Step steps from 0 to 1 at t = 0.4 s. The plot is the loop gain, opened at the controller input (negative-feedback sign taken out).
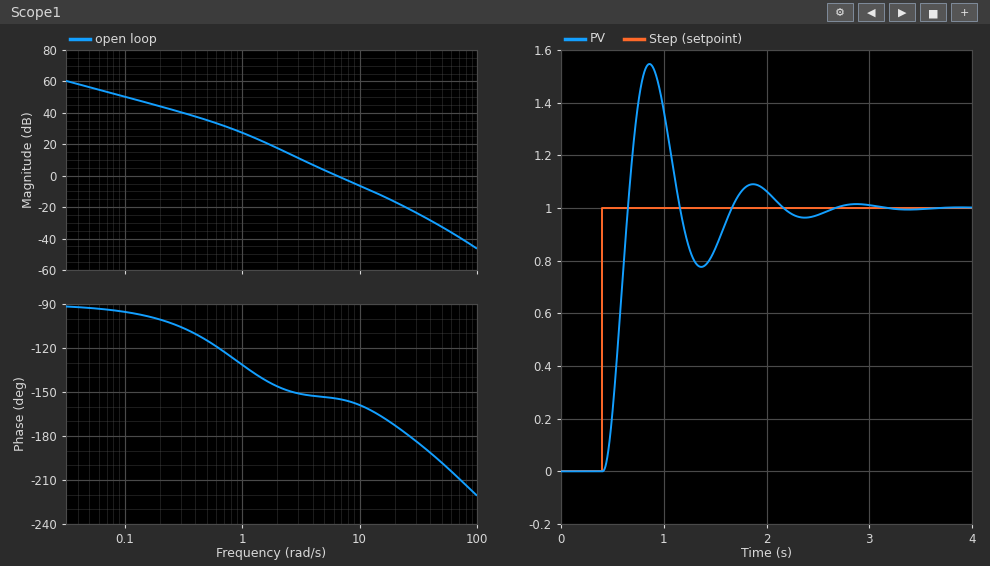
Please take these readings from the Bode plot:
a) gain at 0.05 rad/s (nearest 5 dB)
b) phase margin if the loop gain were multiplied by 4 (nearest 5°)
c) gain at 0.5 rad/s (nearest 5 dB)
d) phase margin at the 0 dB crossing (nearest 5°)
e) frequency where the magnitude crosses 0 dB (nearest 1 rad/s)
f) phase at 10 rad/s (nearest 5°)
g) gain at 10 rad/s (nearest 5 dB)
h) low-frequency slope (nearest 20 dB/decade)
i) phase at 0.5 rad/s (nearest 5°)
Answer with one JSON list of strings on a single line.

["55 dB", "15°", "35 dB", "25°", "6 rad/s", "-160°", "-5 dB", "-20 dB/decade", "-115°"]
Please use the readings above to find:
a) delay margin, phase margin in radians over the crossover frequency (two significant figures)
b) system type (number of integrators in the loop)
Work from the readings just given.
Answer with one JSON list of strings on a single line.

["0.073 s", "1"]
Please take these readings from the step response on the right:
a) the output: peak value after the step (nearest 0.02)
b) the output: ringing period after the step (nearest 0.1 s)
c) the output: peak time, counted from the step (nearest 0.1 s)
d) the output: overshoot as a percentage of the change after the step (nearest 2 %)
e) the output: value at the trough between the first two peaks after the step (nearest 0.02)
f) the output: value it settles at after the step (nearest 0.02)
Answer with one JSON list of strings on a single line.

["1.54", "1.0 s", "0.5 s", "54 %", "0.78", "1.00"]
